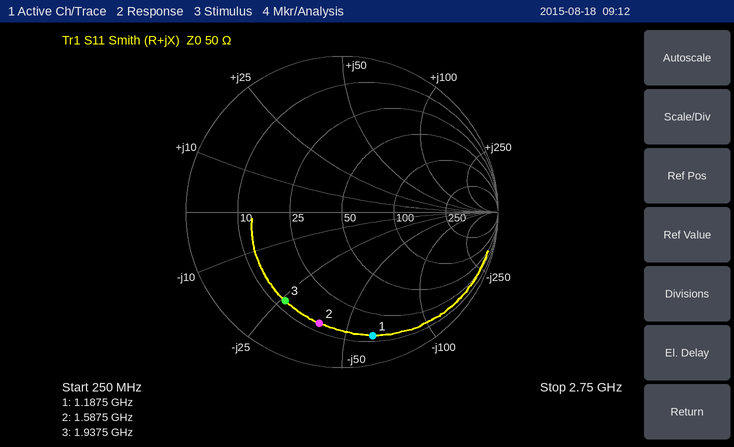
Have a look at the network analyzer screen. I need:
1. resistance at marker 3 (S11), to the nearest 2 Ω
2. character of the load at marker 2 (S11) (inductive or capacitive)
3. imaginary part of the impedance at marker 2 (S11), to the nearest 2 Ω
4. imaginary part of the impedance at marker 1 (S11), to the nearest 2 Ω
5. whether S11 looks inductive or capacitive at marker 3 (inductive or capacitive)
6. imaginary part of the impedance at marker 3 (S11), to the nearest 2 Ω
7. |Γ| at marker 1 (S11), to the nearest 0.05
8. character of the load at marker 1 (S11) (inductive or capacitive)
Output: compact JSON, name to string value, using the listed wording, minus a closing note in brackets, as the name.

{"resistance at marker 3 (S11), to the nearest 2 Ω": "12 Ω", "character of the load at marker 2 (S11)": "capacitive", "imaginary part of the impedance at marker 2 (S11), to the nearest 2 Ω": "-40 Ω", "imaginary part of the impedance at marker 1 (S11), to the nearest 2 Ω": "-62 Ω", "whether S11 looks inductive or capacitive at marker 3": "capacitive", "imaginary part of the impedance at marker 3 (S11), to the nearest 2 Ω": "-26 Ω", "|Γ| at marker 1 (S11), to the nearest 0.05": "0.80", "character of the load at marker 1 (S11)": "capacitive"}
